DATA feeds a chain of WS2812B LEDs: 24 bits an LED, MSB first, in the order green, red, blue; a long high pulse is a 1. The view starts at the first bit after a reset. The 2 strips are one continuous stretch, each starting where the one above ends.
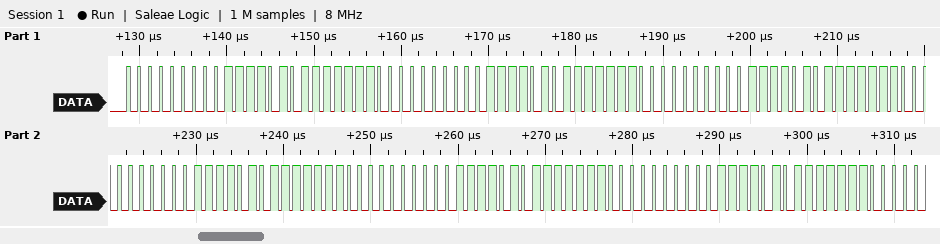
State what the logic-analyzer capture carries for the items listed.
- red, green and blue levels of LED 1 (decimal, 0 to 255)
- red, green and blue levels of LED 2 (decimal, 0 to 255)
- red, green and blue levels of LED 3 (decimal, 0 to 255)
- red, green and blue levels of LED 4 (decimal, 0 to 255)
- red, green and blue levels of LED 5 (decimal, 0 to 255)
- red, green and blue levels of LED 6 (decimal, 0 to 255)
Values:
122, 0, 254
122, 0, 254
122, 0, 254
122, 0, 254
122, 0, 254
122, 0, 254
